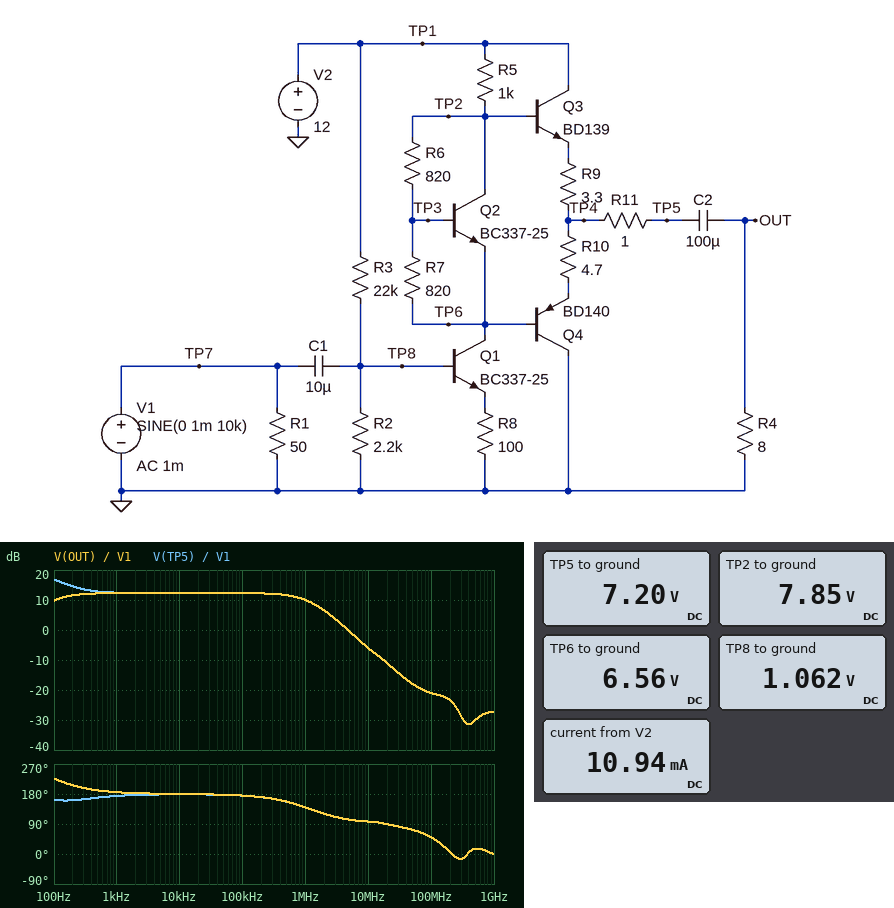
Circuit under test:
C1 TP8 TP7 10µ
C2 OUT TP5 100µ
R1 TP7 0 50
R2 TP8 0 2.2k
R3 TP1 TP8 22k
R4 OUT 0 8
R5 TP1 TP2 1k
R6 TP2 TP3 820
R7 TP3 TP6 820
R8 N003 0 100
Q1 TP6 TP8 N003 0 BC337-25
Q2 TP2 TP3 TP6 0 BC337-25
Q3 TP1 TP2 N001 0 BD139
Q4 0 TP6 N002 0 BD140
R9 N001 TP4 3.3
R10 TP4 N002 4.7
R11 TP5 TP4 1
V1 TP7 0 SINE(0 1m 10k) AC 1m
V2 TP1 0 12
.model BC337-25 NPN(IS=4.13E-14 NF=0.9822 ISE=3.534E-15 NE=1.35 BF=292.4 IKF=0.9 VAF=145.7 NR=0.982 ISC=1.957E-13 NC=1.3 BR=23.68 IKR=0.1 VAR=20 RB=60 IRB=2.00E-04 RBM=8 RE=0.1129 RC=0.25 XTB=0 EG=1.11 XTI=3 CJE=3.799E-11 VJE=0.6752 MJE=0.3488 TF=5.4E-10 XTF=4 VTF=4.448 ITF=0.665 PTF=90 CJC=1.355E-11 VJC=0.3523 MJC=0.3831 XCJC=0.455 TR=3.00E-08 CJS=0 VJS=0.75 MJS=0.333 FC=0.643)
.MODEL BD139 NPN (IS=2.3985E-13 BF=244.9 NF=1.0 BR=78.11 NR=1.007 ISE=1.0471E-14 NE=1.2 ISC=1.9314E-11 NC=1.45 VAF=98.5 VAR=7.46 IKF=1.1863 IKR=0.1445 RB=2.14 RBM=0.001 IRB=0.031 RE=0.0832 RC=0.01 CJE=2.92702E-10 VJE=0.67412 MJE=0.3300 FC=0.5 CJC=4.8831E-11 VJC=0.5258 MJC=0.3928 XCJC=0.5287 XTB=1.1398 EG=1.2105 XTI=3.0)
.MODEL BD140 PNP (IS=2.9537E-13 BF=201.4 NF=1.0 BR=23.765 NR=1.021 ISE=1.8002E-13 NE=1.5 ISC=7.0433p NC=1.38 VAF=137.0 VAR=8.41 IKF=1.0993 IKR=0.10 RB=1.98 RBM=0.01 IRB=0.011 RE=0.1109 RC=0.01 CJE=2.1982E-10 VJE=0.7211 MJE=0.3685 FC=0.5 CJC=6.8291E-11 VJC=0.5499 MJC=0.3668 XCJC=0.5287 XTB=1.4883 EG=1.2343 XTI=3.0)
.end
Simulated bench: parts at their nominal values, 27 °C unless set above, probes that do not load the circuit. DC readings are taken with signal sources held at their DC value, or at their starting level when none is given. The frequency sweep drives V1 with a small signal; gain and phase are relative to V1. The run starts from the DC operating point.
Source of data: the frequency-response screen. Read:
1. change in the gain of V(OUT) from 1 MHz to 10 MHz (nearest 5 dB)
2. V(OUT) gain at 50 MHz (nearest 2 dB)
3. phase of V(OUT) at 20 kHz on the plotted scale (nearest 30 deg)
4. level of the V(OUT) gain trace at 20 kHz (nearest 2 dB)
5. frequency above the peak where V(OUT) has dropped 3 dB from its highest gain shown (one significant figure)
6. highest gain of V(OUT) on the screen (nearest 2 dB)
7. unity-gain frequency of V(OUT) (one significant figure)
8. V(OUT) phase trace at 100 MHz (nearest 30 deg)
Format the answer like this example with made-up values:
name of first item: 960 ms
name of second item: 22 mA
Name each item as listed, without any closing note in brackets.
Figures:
change in the gain of V(OUT) from 1 MHz to 10 MHz: -15 dB
V(OUT) gain at 50 MHz: -18 dB
phase of V(OUT) at 20 kHz on the plotted scale: 180 deg
level of the V(OUT) gain trace at 20 kHz: 12 dB
frequency above the peak where V(OUT) has dropped 3 dB from its highest gain shown: 1 MHz
highest gain of V(OUT) on the screen: 12 dB
unity-gain frequency of V(OUT): 5 MHz
V(OUT) phase trace at 100 MHz: 60 deg
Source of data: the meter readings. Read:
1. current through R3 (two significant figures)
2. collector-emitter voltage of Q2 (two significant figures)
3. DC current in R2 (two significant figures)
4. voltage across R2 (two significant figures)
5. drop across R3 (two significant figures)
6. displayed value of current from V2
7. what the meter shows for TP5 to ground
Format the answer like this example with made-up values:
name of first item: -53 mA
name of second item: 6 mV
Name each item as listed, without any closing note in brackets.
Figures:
current through R3: 500 µA
collector-emitter voltage of Q2: 1.3 V
DC current in R2: 480 µA
voltage across R2: 1.1 V
drop across R3: 11 V
displayed value of current from V2: 10.94 mA
what the meter shows for TP5 to ground: 7.20 V
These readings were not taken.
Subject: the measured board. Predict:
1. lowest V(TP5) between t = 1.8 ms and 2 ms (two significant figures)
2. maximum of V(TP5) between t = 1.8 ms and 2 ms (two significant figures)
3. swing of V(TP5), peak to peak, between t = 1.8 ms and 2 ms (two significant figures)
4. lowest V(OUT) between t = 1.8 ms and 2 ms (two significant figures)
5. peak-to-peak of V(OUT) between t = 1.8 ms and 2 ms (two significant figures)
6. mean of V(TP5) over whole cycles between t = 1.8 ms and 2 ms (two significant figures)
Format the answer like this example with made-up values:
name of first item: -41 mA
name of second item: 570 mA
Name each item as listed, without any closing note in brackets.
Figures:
lowest V(TP5) between t = 1.8 ms and 2 ms: 7.2 V
maximum of V(TP5) between t = 1.8 ms and 2 ms: 7.2 V
swing of V(TP5), peak to peak, between t = 1.8 ms and 2 ms: 8.3 mV
lowest V(OUT) between t = 1.8 ms and 2 ms: -4.1 mV
peak-to-peak of V(OUT) between t = 1.8 ms and 2 ms: 8.3 mV
mean of V(TP5) over whole cycles between t = 1.8 ms and 2 ms: 7.2 V
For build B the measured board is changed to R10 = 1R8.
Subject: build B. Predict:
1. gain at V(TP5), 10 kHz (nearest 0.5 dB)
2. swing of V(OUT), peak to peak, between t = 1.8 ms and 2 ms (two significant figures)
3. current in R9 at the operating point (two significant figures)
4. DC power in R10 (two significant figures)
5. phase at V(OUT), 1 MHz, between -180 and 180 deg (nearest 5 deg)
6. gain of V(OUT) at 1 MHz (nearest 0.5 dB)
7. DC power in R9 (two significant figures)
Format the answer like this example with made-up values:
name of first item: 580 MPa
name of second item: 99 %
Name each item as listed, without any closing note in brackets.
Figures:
gain at V(TP5), 10 kHz: 13.0 dB
swing of V(OUT), peak to peak, between t = 1.8 ms and 2 ms: 8.8 mV
current in R9 at the operating point: 7.7 mA
DC power in R10: 110 µW
phase at V(OUT), 1 MHz, between -180 and 180 deg: 145 deg
gain of V(OUT) at 1 MHz: 11.0 dB
DC power in R9: 200 µW
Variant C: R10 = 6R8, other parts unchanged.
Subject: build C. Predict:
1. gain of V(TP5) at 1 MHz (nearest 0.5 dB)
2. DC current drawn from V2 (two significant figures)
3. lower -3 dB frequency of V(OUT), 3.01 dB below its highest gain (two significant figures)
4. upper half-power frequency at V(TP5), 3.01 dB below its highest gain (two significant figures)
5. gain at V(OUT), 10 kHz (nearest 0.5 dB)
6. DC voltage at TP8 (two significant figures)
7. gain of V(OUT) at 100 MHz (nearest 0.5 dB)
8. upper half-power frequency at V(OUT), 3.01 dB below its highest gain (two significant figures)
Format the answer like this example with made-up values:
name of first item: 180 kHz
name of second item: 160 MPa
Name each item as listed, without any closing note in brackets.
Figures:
gain of V(TP5) at 1 MHz: 9.5 dB
DC current drawn from V2: 10 mA
lower -3 dB frequency of V(OUT), 3.01 dB below its highest gain: 85 Hz
upper half-power frequency at V(TP5), 3.01 dB below its highest gain: 130 Hz
gain at V(OUT), 10 kHz: 12.0 dB
DC voltage at TP8: 1.1 V
gain of V(OUT) at 100 MHz: -21.5 dB
upper half-power frequency at V(OUT), 3.01 dB below its highest gain: 1.1 MHz
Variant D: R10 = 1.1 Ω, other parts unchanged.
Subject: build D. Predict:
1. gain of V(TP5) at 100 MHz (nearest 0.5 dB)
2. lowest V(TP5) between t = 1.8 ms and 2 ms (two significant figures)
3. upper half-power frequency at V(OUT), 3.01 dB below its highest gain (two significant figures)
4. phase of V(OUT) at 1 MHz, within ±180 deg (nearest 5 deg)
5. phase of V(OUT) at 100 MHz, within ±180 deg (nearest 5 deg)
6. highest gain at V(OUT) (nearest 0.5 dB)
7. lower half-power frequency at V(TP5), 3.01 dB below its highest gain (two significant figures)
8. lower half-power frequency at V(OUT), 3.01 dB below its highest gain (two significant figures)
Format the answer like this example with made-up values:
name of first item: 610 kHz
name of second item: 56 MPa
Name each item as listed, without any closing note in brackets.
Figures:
gain of V(TP5) at 100 MHz: -19.5 dB
lowest V(TP5) between t = 1.8 ms and 2 ms: 7.2 V
upper half-power frequency at V(OUT), 3.01 dB below its highest gain: 1.4 MHz
phase of V(OUT) at 1 MHz, within ±180 deg: 145 deg
phase of V(OUT) at 100 MHz, within ±180 deg: 45 deg
highest gain at V(OUT): 13.0 dB
lower half-power frequency at V(TP5), 3.01 dB below its highest gain: 7.4 Hz
lower half-power frequency at V(OUT), 3.01 dB below its highest gain: 95 Hz
